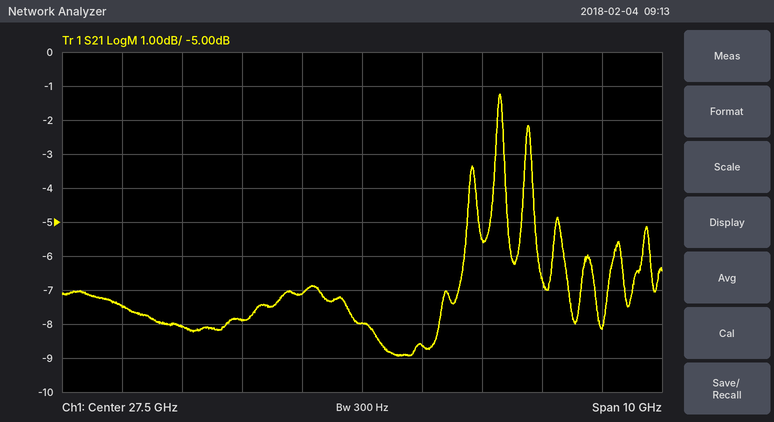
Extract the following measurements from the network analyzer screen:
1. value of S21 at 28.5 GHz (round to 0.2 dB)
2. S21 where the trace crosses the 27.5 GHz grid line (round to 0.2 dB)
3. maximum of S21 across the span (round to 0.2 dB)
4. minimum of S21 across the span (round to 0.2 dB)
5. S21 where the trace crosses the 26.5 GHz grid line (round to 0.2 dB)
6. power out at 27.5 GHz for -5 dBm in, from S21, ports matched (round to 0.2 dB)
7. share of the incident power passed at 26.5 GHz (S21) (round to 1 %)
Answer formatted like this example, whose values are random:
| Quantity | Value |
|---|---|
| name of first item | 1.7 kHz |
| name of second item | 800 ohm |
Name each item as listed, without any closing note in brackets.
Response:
| Quantity | Value |
|---|---|
| value of S21 at 28.5 GHz | -8.6 dB |
| S21 where the trace crosses the 27.5 GHz grid line | -8.0 dB |
| maximum of S21 across the span | -1.2 dB |
| minimum of S21 across the span | -9.0 dB |
| S21 where the trace crosses the 26.5 GHz grid line | -7.2 dB |
| power out at 27.5 GHz for -5 dBm in, from S21, ports matched | -13.0 dBm |
| share of the incident power passed at 26.5 GHz (S21) | 19 % |
